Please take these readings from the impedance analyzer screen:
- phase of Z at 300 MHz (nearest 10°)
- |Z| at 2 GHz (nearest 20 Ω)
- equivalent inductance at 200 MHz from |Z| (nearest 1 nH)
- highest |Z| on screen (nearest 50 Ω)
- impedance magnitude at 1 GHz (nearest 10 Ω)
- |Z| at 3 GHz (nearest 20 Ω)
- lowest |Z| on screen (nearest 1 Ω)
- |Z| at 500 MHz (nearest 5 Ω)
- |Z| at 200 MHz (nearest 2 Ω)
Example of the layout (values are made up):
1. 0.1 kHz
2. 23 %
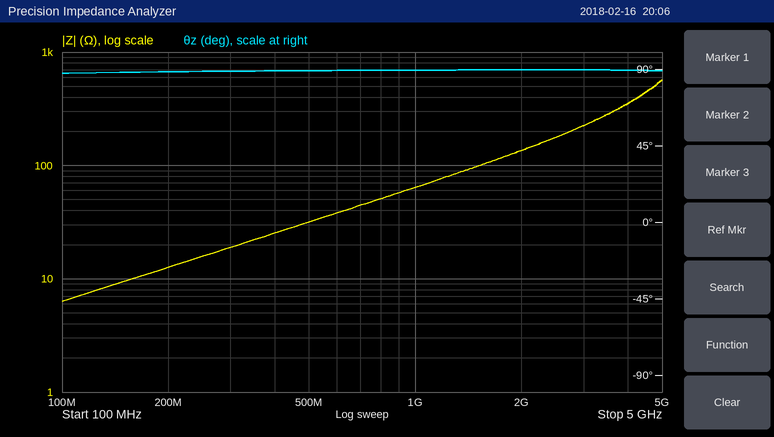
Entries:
1. 90°
2. 140 Ω
3. 10 nH
4. 550 Ω
5. 60 Ω
6. 220 Ω
7. 6 Ω
8. 30 Ω
9. 12 Ω
